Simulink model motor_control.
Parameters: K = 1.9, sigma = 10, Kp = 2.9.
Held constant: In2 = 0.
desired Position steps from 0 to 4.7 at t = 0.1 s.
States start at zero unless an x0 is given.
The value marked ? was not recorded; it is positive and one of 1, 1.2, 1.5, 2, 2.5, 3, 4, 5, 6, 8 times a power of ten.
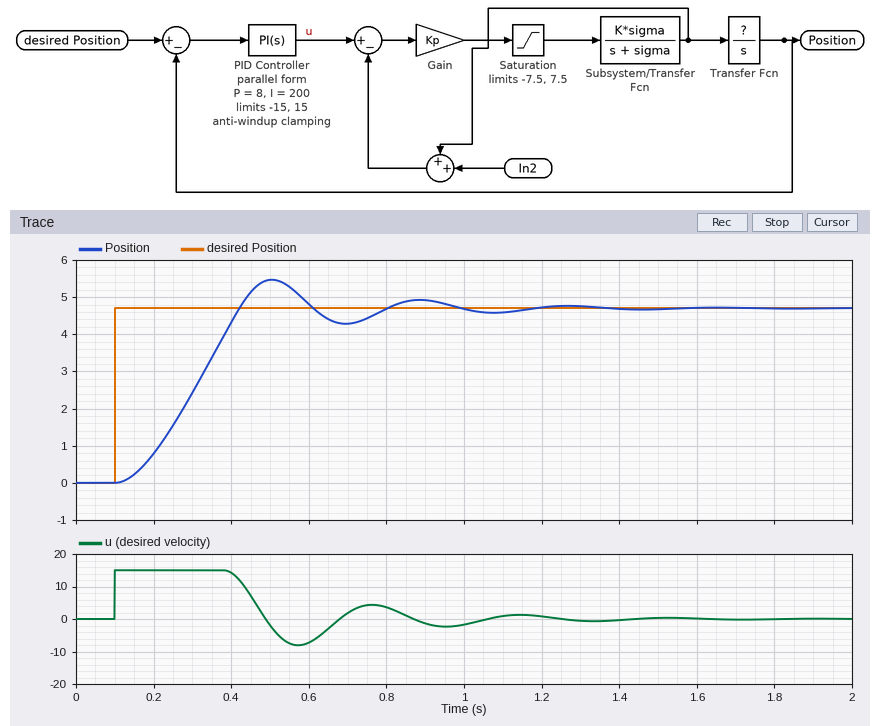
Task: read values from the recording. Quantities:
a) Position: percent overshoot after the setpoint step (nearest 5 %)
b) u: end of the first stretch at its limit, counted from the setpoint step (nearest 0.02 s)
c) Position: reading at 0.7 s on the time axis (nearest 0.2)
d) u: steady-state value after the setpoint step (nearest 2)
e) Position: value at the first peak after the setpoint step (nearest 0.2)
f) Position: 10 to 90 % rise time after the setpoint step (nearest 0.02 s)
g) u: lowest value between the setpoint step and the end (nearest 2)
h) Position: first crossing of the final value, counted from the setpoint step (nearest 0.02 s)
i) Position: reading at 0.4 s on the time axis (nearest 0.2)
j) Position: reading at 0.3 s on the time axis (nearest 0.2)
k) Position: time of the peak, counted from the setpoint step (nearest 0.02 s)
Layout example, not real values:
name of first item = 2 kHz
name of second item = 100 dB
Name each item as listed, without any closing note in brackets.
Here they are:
Position: percent overshoot after the setpoint step = 15 %
u: end of the first stretch at its limit, counted from the setpoint step = 0.30 s
Position: reading at 0.7 s on the time axis = 4.2
u: steady-state value after the setpoint step = 0
Position: value at the first peak after the setpoint step = 5.4
Position: 10 to 90 % rise time after the setpoint step = 0.22 s
u: lowest value between the setpoint step and the end = -8
Position: first crossing of the final value, counted from the setpoint step = 0.32 s
Position: reading at 0.4 s on the time axis = 4.4
Position: reading at 0.3 s on the time axis = 2.4
Position: time of the peak, counted from the setpoint step = 0.40 s
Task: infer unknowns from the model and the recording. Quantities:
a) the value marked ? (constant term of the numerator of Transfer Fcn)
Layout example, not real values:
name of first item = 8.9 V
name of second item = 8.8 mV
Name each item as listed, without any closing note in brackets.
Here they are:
the value marked ? = 1.5
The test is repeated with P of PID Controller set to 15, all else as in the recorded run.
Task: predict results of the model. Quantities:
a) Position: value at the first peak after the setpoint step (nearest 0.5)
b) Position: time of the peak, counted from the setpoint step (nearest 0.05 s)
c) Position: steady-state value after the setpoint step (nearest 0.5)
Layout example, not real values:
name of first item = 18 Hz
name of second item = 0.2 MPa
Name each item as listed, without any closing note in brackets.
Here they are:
Position: value at the first peak after the setpoint step = 5.0
Position: time of the peak, counted from the setpoint step = 0.40 s
Position: steady-state value after the setpoint step = 4.5
